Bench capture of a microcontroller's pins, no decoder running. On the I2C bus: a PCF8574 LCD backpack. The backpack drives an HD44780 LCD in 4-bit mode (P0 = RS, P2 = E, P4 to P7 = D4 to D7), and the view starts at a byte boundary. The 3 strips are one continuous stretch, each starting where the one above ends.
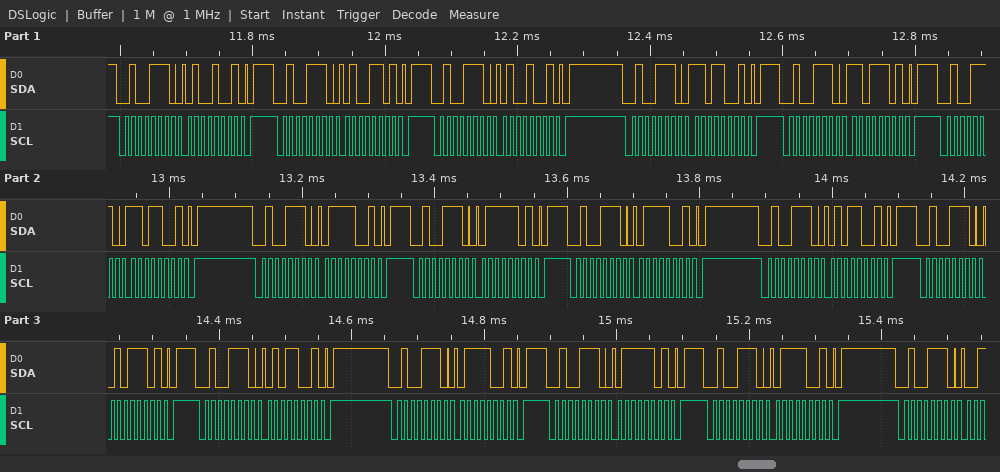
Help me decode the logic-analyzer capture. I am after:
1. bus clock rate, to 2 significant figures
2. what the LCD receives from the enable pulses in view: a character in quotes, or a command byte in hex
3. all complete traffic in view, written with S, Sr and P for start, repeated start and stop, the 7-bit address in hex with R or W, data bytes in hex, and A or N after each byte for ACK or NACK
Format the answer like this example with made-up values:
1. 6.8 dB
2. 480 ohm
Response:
1. 100 kHz
2. 'M' 'u'
3. S 27W A 49 A P S 27W A 4D A P S 27W A 49 A P S 27W A D9 A P S 27W A DD A P S 27W A D9 A P S 27W A 79 A P S 27W A 7D A P S 27W A 79 A P S 27W A 59 A P S 27W A 5D A P S 27W A 59 A P S 27W A 79 A P S 27W A 7D A P S 27W A 79 A P S 27W A
